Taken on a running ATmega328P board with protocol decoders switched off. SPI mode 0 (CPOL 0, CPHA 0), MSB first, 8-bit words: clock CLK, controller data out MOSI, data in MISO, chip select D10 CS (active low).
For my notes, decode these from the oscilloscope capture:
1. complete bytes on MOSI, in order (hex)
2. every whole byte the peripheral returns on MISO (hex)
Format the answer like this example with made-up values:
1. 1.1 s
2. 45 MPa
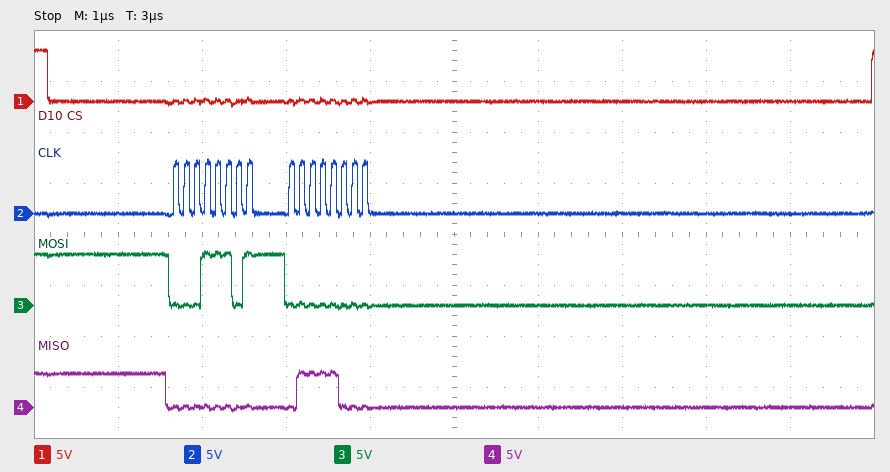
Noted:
1. 1D 00
2. 00 78
